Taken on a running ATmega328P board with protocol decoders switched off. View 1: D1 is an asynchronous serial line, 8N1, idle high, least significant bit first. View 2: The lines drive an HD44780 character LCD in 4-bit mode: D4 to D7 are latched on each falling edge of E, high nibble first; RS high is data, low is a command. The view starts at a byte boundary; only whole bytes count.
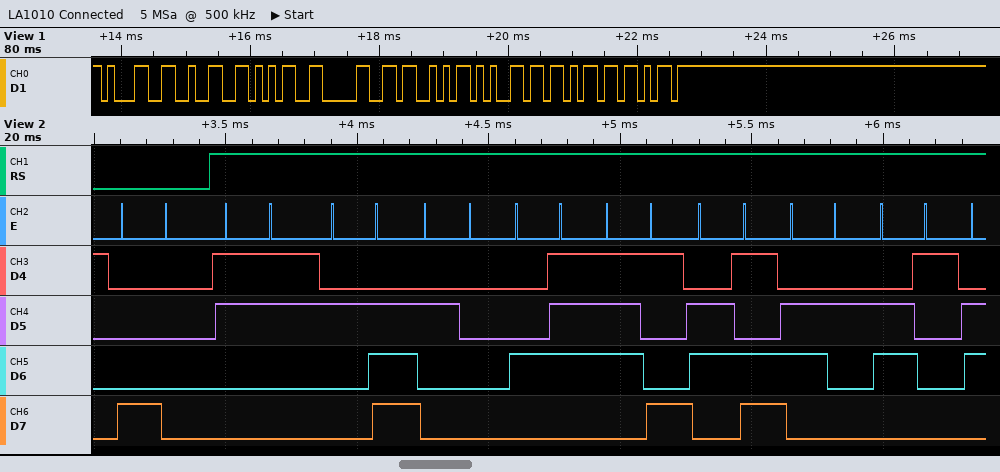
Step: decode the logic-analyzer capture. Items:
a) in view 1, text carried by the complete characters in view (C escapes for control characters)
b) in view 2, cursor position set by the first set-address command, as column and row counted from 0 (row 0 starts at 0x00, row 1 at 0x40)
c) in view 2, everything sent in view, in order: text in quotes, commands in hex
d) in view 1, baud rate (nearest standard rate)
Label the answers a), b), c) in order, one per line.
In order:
a) "1250Sekk"
b) column 0, row 0
c) 0x80 "3. Gymba"
d) 9600 baud
